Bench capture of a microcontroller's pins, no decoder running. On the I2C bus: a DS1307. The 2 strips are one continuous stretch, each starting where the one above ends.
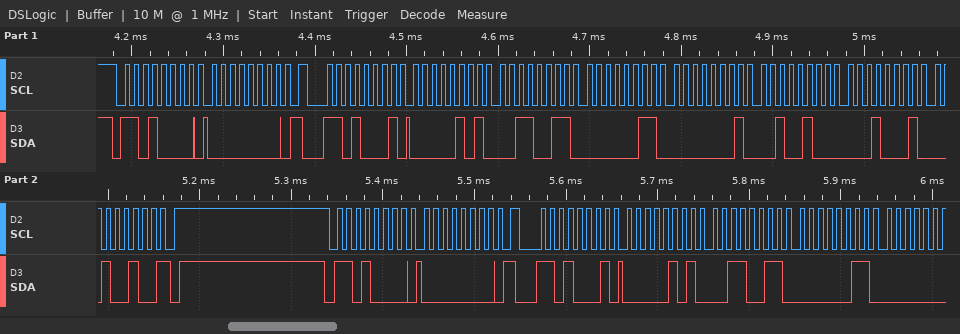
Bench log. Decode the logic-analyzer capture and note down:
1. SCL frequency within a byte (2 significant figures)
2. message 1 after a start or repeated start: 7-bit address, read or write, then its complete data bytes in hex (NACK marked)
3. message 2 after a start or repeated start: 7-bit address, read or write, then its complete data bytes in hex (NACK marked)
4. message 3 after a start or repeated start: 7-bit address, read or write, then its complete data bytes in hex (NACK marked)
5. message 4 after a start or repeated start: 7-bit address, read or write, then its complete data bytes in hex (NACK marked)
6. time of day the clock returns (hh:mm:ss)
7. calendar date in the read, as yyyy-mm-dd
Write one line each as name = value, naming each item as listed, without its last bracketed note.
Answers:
SCL frequency within a byte = 100 kHz
message 1 after a start or repeated start: 7-bit address, read or write, then its complete data bytes in hex = 0x68 write: 00
message 2 after a start or repeated start: 7-bit address, read or write, then its complete data bytes in hex = 0x68 read: 05 33 03 01 24 11 24 NACK
message 3 after a start or repeated start: 7-bit address, read or write, then its complete data bytes in hex = 0x68 write: 00
message 4 after a start or repeated start: 7-bit address, read or write, then its complete data bytes in hex = 0x68 read: 05 33 03
time of day the clock returns = 03:33:05
calendar date in the read, as yyyy-mm-dd = 2024-11-24
